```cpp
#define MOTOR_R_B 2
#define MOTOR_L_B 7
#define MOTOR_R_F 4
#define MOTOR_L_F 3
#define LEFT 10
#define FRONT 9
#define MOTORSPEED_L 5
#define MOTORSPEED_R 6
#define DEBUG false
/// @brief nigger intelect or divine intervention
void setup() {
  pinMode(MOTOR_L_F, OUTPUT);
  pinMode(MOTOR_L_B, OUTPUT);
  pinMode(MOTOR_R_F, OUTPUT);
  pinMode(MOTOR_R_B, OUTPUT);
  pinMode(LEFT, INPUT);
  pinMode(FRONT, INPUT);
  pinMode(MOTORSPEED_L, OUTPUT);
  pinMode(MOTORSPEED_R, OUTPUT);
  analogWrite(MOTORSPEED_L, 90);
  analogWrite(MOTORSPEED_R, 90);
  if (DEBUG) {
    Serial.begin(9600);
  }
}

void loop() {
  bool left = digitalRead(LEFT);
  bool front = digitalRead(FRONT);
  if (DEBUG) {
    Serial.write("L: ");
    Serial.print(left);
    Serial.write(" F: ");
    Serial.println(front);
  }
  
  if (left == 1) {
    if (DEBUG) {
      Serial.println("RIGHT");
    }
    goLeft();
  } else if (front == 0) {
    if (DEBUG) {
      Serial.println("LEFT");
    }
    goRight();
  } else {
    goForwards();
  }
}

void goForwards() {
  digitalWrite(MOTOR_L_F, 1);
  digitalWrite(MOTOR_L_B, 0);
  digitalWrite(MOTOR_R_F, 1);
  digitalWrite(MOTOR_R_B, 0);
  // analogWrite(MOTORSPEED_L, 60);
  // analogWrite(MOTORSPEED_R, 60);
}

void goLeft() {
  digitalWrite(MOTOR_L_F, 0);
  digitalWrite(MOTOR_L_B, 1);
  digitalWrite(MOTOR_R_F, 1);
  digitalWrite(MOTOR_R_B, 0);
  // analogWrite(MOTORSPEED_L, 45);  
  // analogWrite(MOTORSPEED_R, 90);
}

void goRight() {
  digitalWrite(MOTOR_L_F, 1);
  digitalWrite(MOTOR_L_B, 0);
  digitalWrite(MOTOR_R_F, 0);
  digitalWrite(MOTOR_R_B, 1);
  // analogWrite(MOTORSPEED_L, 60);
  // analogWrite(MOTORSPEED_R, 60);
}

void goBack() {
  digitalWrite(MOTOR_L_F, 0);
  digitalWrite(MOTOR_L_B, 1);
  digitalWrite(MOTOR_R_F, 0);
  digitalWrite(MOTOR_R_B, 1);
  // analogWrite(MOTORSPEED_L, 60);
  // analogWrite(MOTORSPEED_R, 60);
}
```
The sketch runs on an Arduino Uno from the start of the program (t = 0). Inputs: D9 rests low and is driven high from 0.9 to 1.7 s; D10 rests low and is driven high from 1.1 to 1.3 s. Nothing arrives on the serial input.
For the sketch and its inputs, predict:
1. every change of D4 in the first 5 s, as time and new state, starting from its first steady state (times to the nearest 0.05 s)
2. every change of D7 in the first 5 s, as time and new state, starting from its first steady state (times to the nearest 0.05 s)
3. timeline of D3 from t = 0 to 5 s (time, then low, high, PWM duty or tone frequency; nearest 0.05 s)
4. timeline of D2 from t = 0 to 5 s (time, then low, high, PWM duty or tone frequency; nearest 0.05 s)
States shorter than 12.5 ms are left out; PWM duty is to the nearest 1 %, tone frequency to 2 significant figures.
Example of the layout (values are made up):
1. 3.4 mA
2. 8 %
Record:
1. 0 s low; 0.9 s high; 1.7 s low
2. 0 s low; 1.1 s high; 1.3 s low
3. 0 s high; 1.1 s low; 1.3 s high
4. 0 s high; 0.9 s low; 1.7 s high
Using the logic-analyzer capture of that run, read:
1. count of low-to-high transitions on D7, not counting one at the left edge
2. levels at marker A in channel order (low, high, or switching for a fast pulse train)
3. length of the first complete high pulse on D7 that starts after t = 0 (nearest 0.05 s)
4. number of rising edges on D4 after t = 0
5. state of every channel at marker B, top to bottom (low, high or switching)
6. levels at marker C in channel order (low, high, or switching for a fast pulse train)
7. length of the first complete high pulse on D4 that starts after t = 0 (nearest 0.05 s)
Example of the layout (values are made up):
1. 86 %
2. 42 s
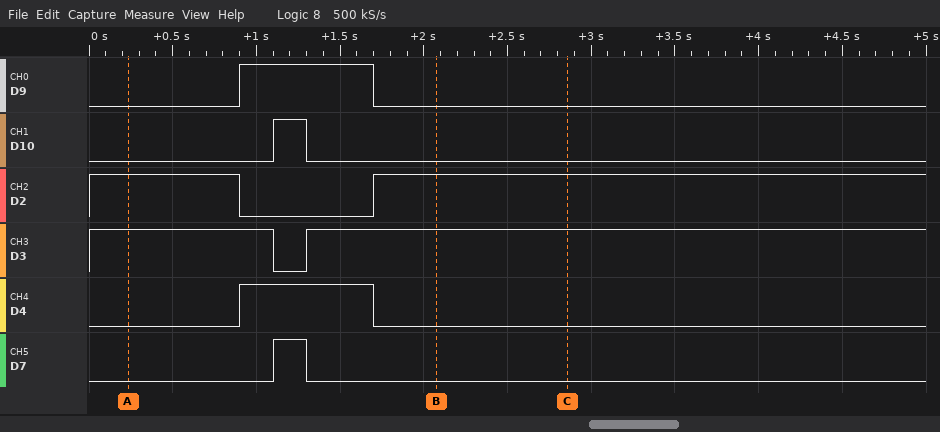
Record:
1. 1
2. D9 low, D10 low, D2 high, D3 high, D4 low, D7 low
3. 0.20 s
4. 1
5. D9 low, D10 low, D2 high, D3 high, D4 low, D7 low
6. D9 low, D10 low, D2 high, D3 high, D4 low, D7 low
7. 0.80 s
